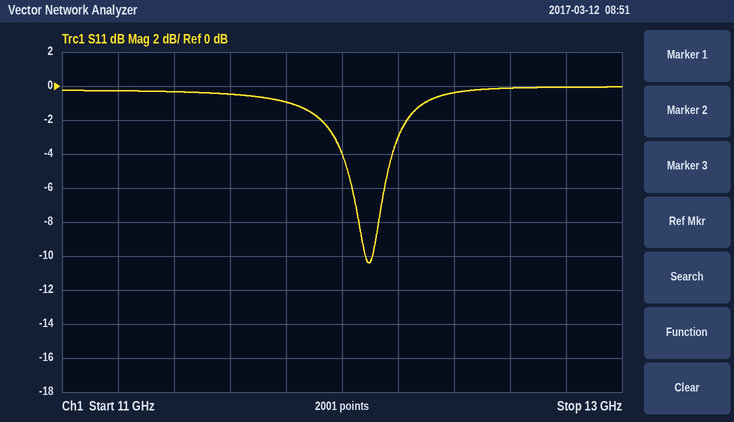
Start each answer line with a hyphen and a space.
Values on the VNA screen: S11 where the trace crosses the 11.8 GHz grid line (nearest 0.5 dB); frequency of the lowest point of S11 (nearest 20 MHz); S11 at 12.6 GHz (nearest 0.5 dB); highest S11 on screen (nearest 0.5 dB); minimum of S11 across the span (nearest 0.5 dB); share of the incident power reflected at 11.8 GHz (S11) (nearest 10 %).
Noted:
- -1.0 dB
- 12.10 GHz
- 0.0 dB
- 0.0 dB
- -10.5 dB
- 80 %
